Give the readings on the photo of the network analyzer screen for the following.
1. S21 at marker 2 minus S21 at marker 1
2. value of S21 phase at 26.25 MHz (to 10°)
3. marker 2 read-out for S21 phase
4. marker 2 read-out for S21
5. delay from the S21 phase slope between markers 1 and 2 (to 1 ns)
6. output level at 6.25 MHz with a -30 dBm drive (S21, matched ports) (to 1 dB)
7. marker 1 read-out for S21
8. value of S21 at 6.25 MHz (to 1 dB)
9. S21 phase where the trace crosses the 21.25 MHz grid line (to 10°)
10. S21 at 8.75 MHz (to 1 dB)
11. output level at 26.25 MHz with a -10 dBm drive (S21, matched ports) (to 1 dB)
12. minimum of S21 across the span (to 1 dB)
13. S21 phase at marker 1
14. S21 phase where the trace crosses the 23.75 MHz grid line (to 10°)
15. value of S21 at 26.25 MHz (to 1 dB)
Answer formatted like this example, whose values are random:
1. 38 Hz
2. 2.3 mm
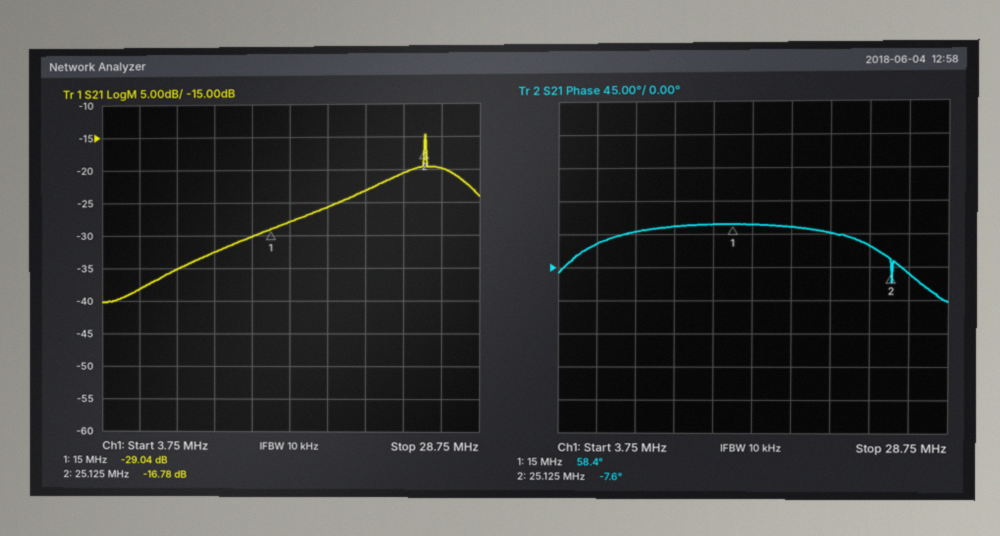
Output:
1. 12.26 dB
2. -10°
3. -7.6°
4. -16.78 dB
5. 18 ns
6. -68 dBm
7. -29.04 dB
8. -38 dB
9. 50°
10. -35 dB
11. -30 dBm
12. -40 dB
13. 58.4°
14. 30°
15. -20 dB
